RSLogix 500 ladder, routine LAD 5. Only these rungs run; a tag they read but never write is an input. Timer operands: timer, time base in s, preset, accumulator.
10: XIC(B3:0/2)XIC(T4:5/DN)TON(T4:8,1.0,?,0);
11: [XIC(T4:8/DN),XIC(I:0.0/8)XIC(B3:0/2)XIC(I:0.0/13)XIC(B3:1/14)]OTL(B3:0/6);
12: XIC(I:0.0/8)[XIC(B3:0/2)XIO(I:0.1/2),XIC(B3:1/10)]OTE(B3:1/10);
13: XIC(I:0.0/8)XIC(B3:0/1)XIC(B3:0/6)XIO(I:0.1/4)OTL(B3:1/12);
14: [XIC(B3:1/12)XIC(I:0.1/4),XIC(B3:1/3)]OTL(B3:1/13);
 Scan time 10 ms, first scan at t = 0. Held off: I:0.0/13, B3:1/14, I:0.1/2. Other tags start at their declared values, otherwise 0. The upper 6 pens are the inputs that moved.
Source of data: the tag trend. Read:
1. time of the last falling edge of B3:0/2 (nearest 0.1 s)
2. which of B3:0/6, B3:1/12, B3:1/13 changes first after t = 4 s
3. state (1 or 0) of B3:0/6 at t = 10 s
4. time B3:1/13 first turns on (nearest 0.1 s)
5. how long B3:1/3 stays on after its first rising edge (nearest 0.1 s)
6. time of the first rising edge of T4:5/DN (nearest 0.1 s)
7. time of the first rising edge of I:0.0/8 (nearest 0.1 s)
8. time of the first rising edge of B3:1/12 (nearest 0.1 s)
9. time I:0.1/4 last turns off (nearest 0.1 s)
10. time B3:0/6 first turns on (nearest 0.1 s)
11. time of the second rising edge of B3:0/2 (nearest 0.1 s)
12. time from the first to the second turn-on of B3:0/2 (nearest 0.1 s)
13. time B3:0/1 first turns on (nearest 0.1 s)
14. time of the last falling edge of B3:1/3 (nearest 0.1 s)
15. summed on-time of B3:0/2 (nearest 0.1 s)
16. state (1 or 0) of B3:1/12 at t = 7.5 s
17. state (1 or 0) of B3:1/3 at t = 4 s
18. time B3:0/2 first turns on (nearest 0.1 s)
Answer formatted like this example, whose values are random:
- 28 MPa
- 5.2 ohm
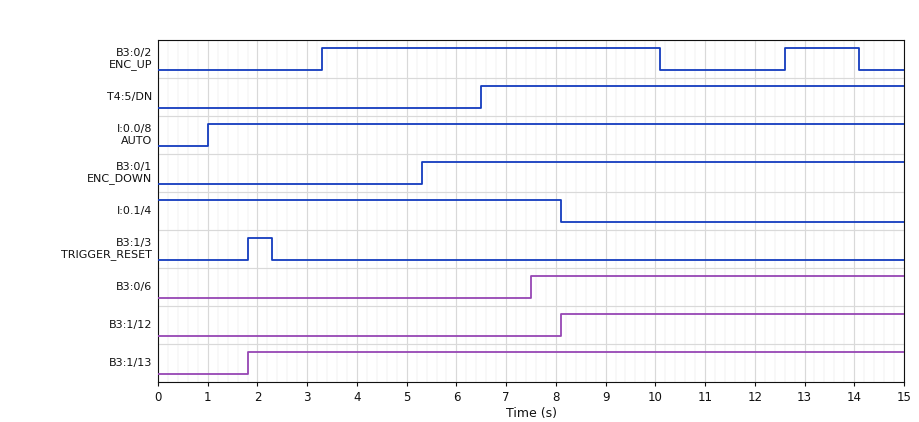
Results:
- 14.1 s
- B3:0/6
- 1
- 1.8 s
- 0.5 s
- 6.5 s
- 1.0 s
- 8.1 s
- 8.1 s
- 7.5 s
- 12.6 s
- 9.3 s
- 5.3 s
- 2.3 s
- 8.3 s
- 0
- 0
- 3.3 s
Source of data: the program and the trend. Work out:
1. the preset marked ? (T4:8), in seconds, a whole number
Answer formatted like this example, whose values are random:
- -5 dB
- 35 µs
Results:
- 1 s
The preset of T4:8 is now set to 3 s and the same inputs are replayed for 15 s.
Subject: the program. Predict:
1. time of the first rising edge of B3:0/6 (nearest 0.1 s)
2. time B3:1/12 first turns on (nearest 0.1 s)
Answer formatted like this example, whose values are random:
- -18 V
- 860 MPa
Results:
- 9.5 s
- 9.5 s
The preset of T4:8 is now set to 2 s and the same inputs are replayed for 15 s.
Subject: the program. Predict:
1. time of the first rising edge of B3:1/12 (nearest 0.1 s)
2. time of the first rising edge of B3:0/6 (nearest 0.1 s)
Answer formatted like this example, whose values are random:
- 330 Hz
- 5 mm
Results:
- 8.5 s
- 8.5 s
